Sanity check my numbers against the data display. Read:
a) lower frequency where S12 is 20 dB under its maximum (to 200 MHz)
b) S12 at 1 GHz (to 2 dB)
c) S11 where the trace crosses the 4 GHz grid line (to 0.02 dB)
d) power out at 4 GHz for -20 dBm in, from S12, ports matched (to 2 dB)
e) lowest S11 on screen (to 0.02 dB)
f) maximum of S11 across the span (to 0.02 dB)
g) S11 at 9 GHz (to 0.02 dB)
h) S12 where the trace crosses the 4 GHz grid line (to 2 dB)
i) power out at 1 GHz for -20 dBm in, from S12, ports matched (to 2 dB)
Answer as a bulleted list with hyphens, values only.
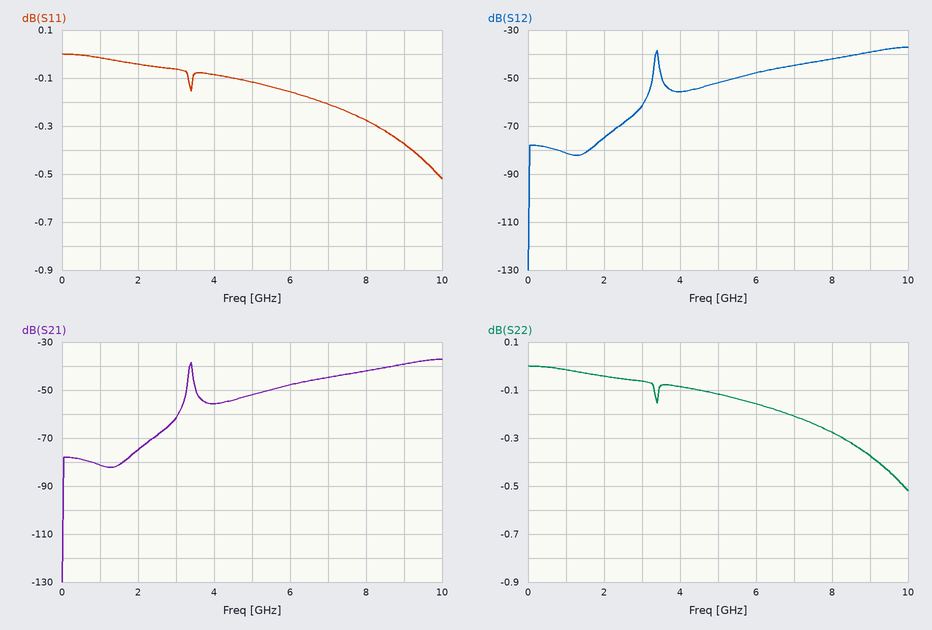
- 3.2 GHz
- -82 dB
- -0.08 dB
- -76 dBm
- -0.52 dB
- 0.00 dB
- -0.38 dB
- -56 dB
- -102 dBm
